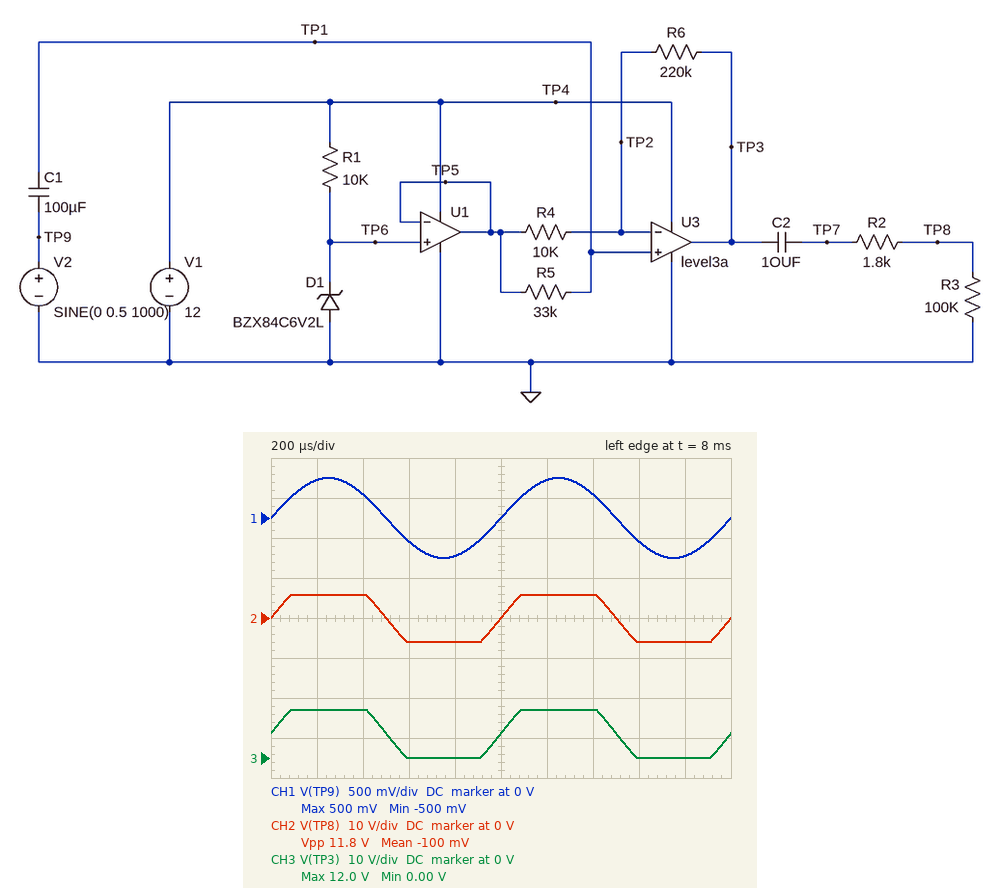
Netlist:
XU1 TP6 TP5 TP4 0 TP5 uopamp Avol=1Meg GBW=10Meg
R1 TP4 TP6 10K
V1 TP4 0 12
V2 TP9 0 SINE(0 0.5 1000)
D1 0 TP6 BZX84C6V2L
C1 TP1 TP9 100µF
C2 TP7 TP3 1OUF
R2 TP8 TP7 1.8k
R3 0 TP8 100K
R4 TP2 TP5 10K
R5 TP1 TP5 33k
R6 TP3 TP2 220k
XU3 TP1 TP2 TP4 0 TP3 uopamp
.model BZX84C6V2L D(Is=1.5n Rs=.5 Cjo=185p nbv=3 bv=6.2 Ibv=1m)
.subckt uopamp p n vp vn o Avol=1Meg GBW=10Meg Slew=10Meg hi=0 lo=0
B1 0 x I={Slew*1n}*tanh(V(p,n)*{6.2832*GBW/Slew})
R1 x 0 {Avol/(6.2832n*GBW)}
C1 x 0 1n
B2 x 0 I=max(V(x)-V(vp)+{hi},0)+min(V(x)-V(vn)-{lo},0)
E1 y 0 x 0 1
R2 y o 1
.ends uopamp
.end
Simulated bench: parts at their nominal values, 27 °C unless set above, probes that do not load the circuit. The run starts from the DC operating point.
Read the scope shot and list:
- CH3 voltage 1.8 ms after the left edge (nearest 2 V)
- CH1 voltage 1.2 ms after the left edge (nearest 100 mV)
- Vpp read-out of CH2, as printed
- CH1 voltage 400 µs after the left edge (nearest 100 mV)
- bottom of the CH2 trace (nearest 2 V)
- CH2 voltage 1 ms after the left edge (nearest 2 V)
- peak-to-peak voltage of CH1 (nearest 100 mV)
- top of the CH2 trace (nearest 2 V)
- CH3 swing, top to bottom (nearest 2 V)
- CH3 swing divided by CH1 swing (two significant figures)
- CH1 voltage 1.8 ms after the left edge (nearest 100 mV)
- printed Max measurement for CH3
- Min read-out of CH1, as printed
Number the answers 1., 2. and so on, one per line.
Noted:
1. 0 V
2. 500 mV
3. 11.8 V
4. 300 mV
5. -6 V
6. 0 V
7. 1.0 V
8. 6 V
9. 12 V
10. 12
11. -500 mV
12. 12.0 V
13. -500 mV
